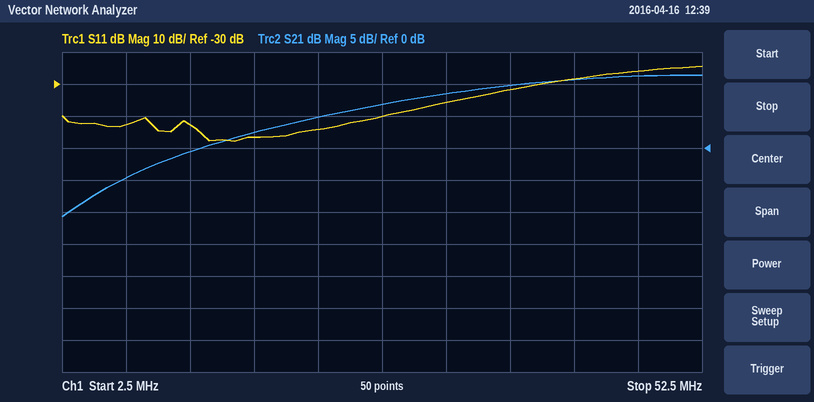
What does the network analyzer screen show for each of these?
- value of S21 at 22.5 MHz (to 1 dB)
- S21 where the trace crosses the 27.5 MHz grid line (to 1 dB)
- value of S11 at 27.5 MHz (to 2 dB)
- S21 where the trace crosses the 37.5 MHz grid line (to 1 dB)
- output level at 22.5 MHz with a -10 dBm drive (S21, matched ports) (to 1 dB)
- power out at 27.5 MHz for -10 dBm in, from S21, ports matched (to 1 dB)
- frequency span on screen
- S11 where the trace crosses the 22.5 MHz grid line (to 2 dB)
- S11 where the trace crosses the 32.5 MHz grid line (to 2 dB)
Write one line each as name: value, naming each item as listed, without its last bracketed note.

value of S21 at 22.5 MHz: 5 dB
S21 where the trace crosses the 27.5 MHz grid line: 7 dB
value of S11 at 27.5 MHz: -40 dB
S21 where the trace crosses the 37.5 MHz grid line: 10 dB
output level at 22.5 MHz with a -10 dBm drive (S21, matched ports): -5 dBm
power out at 27.5 MHz for -10 dBm in, from S21, ports matched: -3 dBm
frequency span on screen: 50 MHz
S11 where the trace crosses the 22.5 MHz grid line: -44 dB
S11 where the trace crosses the 32.5 MHz grid line: -36 dB
